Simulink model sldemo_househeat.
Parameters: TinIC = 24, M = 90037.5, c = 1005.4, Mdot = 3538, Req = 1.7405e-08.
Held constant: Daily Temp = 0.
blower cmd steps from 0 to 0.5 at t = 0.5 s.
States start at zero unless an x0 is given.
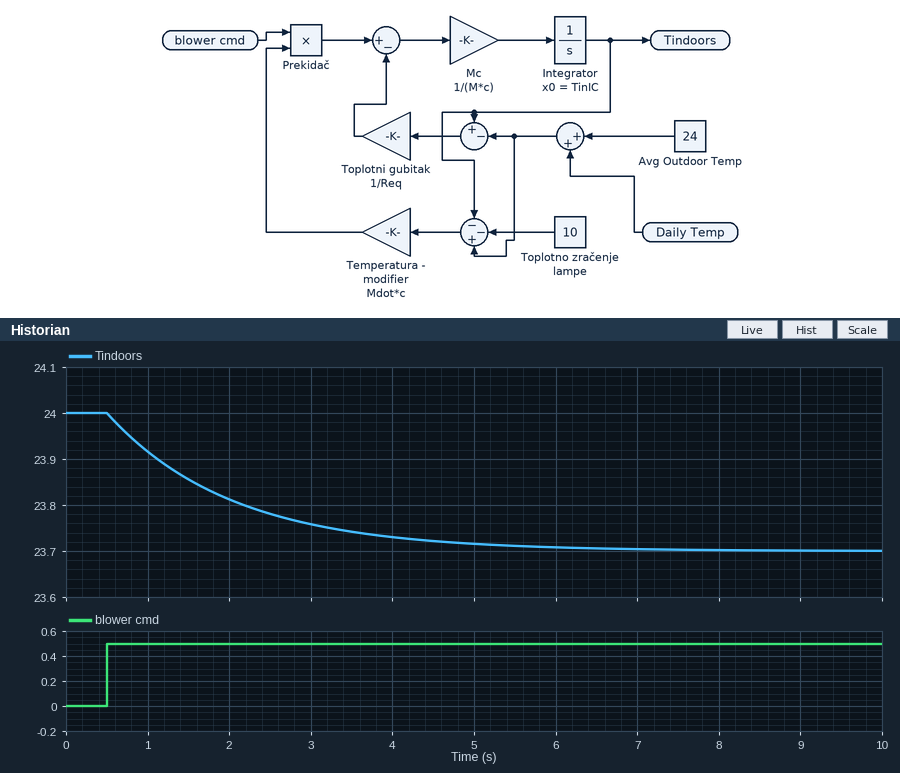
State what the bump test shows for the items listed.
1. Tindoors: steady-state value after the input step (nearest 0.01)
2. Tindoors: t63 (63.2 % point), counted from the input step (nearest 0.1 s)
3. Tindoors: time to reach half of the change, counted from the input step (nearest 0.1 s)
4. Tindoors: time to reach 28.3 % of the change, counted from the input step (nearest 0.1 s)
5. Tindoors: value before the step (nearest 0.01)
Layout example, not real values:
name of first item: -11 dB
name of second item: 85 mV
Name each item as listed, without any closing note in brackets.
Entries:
Tindoors: steady-state value after the input step: 23.70
Tindoors: t63 (63.2 % point), counted from the input step: 1.5 s
Tindoors: time to reach half of the change, counted from the input step: 1.1 s
Tindoors: time to reach 28.3 % of the change, counted from the input step: 0.5 s
Tindoors: value before the step: 24.00
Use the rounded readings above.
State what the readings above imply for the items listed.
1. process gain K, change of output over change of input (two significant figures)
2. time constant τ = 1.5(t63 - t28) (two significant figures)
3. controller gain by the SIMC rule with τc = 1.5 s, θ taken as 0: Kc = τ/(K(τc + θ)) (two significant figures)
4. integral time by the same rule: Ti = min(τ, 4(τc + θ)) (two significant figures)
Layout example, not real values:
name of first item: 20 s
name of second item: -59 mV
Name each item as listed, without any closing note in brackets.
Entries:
process gain K, change of output over change of input: -0.60
time constant τ = 1.5(t63 - t28): 1.5 s
controller gain by the SIMC rule with τc = 1.5 s, θ taken as 0: Kc = τ/(K(τc + θ)): -1.7
integral time by the same rule: Ti = min(τ, 4(τc + θ)): 1.5 s
